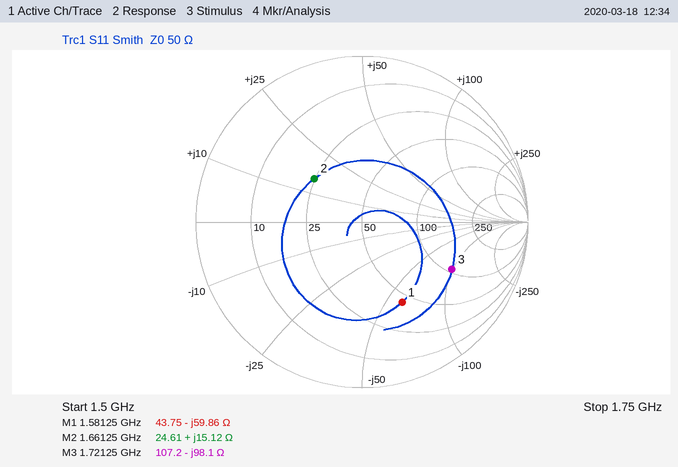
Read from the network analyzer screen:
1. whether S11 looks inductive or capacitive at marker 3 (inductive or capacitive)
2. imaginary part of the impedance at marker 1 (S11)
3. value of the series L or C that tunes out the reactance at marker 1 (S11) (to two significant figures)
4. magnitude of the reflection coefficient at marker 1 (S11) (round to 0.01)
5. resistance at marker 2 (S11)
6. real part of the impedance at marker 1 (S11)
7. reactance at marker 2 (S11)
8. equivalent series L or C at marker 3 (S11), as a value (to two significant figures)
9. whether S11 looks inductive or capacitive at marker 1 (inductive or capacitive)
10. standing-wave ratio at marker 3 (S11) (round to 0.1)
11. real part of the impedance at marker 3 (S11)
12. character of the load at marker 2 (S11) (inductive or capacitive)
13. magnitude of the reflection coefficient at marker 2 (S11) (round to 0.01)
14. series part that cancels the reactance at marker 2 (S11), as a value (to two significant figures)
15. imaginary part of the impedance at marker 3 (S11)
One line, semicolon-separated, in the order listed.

capacitive; -59.86 Ω; 6.0 nH; 0.54; 24.61 Ω; 43.75 Ω; +15.12 Ω; 940 fF; capacitive; 4.2; 107.2 Ω; inductive; 0.39; 6.3 pF; -98.1 Ω
